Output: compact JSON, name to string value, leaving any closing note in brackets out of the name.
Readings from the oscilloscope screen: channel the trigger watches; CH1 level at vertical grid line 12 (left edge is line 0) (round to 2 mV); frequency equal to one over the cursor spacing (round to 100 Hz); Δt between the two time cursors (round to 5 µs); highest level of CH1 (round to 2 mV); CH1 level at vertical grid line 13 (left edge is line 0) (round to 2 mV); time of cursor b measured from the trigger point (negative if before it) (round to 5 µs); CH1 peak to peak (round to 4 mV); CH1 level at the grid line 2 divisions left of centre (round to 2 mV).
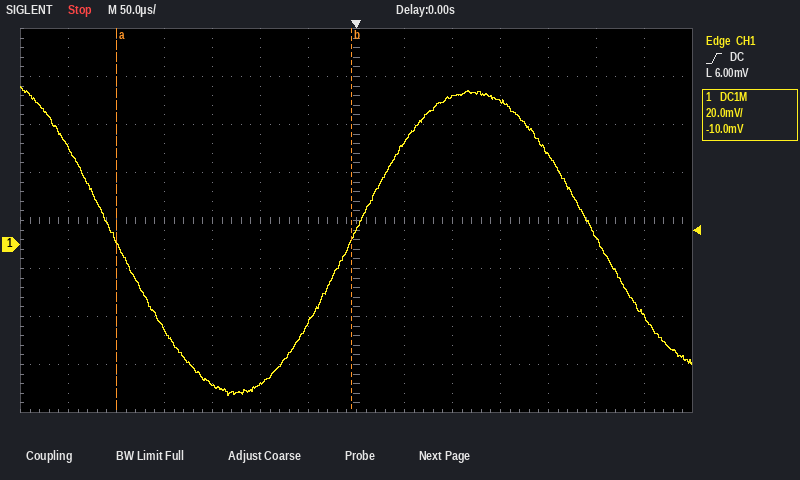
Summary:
{"channel the trigger watches": "CH1", "CH1 level at vertical grid line 12 (left edge is line 0)": "2 mV", "frequency equal to one over the cursor spacing": "4.1 kHz", "Δt between the two time cursors": "245 µs", "highest level of CH1": "66 mV", "CH1 level at vertical grid line 13 (left edge is line 0)": "-30 mV", "time of cursor b measured from the trigger point (negative if before it)": "-5 µs", "CH1 peak to peak": "128 mV", "CH1 level at the grid line 2 divisions left of centre": "-58 mV"}
